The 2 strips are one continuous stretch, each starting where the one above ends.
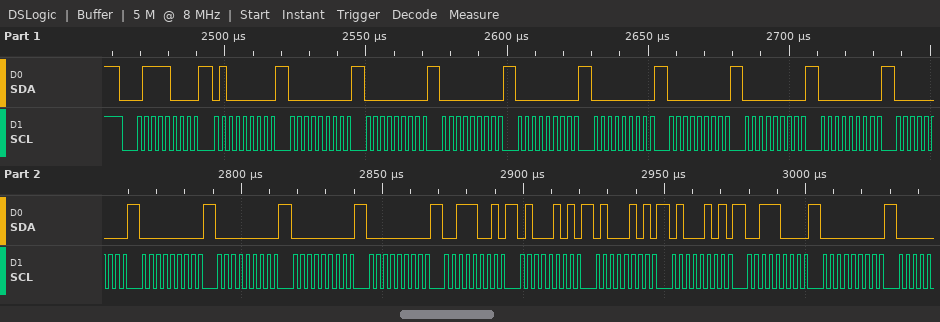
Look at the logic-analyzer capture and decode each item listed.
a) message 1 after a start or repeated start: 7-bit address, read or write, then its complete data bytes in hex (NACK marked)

0x3C write: 40 00 00 00 00 00 00 00 00 00 00 00 00 00 39 45 45 45 38 00
